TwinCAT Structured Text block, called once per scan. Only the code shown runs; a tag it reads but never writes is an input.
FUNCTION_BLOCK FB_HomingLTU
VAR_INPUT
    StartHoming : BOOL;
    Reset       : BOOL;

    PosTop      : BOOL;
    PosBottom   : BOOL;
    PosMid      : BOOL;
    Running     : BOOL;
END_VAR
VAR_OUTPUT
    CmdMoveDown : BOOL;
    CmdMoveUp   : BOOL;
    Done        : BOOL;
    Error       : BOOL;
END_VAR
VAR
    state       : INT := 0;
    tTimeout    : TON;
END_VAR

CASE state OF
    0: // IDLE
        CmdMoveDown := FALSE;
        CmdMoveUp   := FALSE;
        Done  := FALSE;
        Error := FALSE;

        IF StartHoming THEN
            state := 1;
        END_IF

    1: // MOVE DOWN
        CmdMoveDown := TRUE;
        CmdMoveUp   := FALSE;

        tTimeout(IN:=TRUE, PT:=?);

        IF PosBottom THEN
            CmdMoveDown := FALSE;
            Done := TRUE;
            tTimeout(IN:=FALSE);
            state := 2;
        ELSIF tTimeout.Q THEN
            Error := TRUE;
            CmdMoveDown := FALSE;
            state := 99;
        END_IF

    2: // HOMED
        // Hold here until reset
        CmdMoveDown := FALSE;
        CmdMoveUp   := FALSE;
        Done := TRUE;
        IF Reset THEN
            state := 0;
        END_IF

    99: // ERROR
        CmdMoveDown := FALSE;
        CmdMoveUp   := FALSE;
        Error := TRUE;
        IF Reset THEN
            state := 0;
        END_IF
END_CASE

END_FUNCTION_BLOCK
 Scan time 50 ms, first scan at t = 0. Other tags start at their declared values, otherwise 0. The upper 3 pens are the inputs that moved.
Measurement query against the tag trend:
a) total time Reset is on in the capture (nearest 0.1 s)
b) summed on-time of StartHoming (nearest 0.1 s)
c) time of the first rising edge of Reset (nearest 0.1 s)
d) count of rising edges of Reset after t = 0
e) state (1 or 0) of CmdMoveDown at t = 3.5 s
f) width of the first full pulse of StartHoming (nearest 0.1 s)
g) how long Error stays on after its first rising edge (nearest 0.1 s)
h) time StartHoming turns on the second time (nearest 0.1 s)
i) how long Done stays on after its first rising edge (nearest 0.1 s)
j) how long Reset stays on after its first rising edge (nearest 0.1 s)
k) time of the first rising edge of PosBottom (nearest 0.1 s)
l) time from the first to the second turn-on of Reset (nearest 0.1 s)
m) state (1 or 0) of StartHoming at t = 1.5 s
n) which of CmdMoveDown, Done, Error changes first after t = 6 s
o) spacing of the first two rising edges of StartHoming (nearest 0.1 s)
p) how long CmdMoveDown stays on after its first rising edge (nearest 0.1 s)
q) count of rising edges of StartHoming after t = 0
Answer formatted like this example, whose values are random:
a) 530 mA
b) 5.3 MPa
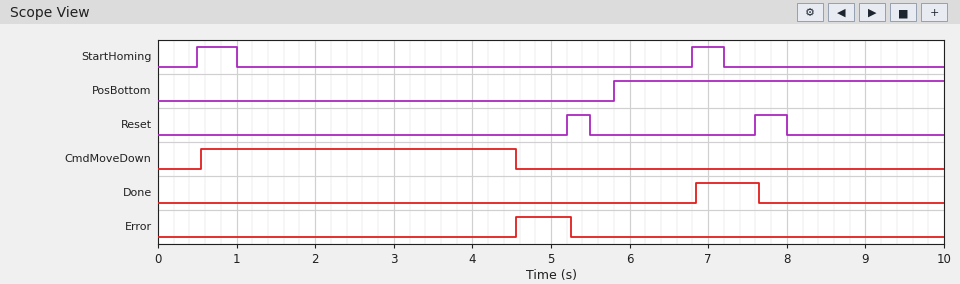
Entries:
a) 0.7 s
b) 0.9 s
c) 5.2 s
d) 2
e) 1
f) 0.5 s
g) 0.7 s
h) 6.8 s
i) 0.8 s
j) 0.3 s
k) 5.8 s
l) 2.4 s
m) 0
n) Done
o) 6.3 s
p) 4.0 s
q) 2
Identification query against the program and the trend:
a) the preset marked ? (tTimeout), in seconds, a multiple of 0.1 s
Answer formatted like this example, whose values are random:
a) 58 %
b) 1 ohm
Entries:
a) 4.0 s
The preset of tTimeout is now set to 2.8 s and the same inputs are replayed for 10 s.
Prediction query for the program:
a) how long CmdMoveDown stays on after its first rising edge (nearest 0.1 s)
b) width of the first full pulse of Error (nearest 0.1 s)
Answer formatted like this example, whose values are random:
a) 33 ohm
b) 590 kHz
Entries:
a) 2.8 s
b) 1.9 s
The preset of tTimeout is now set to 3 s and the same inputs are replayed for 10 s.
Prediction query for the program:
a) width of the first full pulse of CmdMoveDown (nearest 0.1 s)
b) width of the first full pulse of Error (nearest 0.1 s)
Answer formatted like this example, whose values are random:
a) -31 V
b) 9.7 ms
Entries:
a) 3.0 s
b) 1.7 s
